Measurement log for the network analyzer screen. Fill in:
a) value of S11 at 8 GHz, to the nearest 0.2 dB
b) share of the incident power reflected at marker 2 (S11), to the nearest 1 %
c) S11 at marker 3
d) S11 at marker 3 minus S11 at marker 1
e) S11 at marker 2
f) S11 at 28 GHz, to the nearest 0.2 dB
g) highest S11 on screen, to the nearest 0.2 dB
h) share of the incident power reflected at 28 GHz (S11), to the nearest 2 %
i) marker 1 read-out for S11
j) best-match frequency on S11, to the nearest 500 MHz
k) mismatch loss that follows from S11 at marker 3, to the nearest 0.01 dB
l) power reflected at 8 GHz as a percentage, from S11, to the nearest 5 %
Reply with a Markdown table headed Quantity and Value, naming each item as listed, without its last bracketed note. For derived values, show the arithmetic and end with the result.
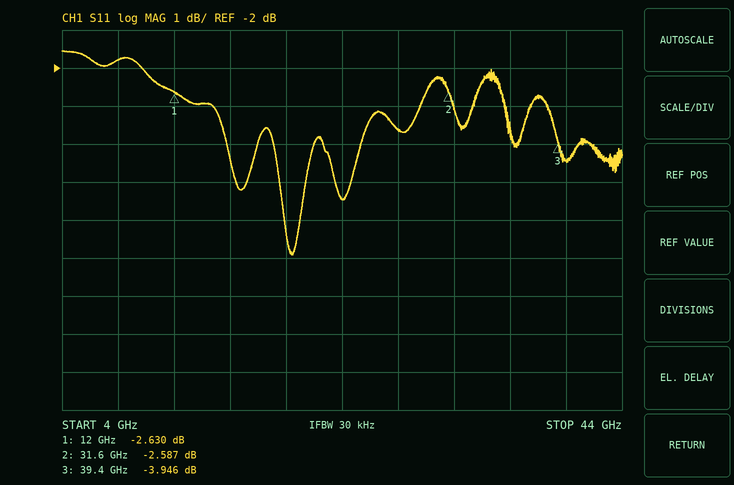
| Quantity | Value |
|---|---|
| value of S11 at 8 GHz, to the nearest 0.2 dB | -1.8 dB |
| share of the incident power reflected at marker 2 (S11), to the nearest 1 % | 10^(-2.587/10) ≈ 55 % |
| S11 at marker 3 | -3.946 dB |
| S11 at marker 3 minus S11 at marker 1 | -3.946 − (-2.63) = -1.316 dB |
| S11 at marker 2 | -2.587 dB |
| S11 at 28 GHz, to the nearest 0.2 dB | -3.6 dB |
| highest S11 on screen, to the nearest 0.2 dB | -1.6 dB |
| share of the incident power reflected at 28 GHz (S11), to the nearest 2 % | 10^(-3.6/10) ≈ 44 % |
| marker 1 read-out for S11 | -2.630 dB |
| best-match frequency on S11, to the nearest 500 MHz | 20.5 GHz |
| mismatch loss that follows from S11 at marker 3, to the nearest 0.01 dB | −10 log10(1 − 10^(-3.946/10)) ≈ 2.24 dB |
| power reflected at 8 GHz as a percentage, from S11, to the nearest 5 % | 10^(-1.8/10) ≈ 66.1 %, so 65 % to the nearest 5 % |
